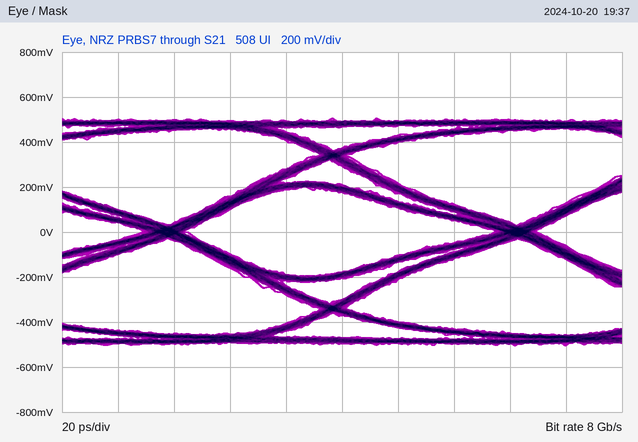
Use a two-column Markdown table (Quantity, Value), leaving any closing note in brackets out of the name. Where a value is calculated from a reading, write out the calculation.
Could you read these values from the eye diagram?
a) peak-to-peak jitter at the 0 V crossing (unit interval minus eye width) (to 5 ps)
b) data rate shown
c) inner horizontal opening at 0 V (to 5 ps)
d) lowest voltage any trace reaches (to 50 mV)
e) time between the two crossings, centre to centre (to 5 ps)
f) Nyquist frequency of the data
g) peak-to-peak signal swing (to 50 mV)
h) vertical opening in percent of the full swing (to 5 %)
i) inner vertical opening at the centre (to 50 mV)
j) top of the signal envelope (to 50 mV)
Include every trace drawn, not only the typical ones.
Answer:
| Quantity | Value |
|---|---|
| peak-to-peak jitter at the 0 V crossing (unit interval minus eye width) | 15 ps |
| data rate shown | 8 Gb/s |
| inner horizontal opening at 0 V | 110 ps |
| lowest voltage any trace reaches | -500 mV |
| time between the two crossings, centre to centre | 125 ps |
| Nyquist frequency of the data | 4 GHz |
| peak-to-peak signal swing | 1.00 V |
| vertical opening in percent of the full swing | 350 mV / 1.00 V ≈ 35 % |
| inner vertical opening at the centre | 350 mV |
| top of the signal envelope | 500 mV |
